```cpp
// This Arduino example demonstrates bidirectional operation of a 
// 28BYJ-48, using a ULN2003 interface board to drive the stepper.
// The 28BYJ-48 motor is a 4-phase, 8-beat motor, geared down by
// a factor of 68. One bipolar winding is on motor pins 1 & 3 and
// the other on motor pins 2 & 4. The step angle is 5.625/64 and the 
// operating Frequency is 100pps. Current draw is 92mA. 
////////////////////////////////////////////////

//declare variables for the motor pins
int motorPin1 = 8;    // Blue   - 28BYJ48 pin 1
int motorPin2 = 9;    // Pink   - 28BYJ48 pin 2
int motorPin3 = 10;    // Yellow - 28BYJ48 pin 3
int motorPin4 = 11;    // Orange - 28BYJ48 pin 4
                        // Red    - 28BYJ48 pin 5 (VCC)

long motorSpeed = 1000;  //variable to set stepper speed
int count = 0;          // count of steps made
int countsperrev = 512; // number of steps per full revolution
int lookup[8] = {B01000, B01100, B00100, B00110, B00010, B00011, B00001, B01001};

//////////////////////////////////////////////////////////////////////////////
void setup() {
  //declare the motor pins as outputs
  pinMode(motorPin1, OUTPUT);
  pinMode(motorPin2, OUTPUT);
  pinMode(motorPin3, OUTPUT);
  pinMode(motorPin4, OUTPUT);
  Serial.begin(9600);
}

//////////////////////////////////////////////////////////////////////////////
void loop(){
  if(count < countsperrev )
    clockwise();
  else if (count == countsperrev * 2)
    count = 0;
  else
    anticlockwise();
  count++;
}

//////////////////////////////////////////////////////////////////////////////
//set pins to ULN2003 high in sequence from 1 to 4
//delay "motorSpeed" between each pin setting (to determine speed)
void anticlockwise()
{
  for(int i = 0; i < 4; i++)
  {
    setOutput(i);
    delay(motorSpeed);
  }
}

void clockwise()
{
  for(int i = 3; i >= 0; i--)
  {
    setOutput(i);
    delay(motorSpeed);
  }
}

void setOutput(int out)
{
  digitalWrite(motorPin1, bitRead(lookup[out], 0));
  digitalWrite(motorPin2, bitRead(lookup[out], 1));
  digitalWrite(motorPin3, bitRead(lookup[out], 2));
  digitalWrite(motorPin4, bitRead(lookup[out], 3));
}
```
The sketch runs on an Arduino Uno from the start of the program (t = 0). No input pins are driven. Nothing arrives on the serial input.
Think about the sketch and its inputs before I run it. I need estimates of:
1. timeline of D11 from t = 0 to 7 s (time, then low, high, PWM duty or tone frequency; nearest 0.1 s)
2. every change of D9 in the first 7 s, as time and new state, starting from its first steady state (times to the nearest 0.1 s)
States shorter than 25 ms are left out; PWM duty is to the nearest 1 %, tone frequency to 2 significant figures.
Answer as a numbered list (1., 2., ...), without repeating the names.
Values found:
1. 0 s low; 2 s high; 4 s low; 6 s high
2. 0 s high; 1 s low; 4 s high; 5 s low
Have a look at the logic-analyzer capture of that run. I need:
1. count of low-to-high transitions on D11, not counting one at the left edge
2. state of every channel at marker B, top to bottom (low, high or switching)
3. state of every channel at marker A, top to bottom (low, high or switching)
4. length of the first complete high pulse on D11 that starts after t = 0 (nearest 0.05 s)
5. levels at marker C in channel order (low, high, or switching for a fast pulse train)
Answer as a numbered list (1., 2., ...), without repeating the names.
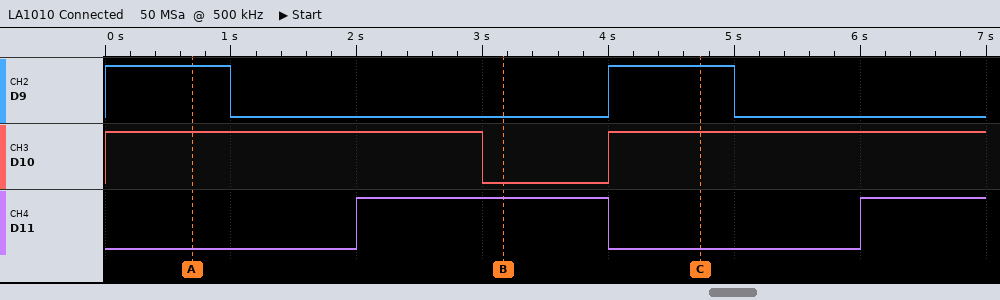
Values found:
1. 2
2. D9 low, D10 low, D11 high
3. D9 high, D10 high, D11 low
4. 2.00 s
5. D9 high, D10 high, D11 low
